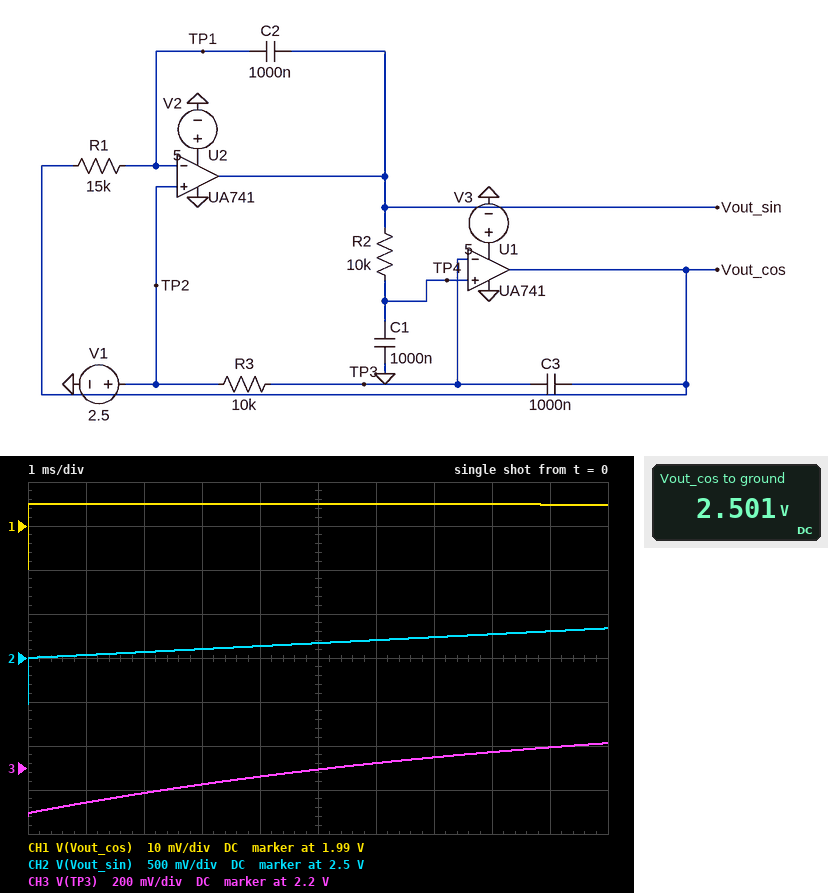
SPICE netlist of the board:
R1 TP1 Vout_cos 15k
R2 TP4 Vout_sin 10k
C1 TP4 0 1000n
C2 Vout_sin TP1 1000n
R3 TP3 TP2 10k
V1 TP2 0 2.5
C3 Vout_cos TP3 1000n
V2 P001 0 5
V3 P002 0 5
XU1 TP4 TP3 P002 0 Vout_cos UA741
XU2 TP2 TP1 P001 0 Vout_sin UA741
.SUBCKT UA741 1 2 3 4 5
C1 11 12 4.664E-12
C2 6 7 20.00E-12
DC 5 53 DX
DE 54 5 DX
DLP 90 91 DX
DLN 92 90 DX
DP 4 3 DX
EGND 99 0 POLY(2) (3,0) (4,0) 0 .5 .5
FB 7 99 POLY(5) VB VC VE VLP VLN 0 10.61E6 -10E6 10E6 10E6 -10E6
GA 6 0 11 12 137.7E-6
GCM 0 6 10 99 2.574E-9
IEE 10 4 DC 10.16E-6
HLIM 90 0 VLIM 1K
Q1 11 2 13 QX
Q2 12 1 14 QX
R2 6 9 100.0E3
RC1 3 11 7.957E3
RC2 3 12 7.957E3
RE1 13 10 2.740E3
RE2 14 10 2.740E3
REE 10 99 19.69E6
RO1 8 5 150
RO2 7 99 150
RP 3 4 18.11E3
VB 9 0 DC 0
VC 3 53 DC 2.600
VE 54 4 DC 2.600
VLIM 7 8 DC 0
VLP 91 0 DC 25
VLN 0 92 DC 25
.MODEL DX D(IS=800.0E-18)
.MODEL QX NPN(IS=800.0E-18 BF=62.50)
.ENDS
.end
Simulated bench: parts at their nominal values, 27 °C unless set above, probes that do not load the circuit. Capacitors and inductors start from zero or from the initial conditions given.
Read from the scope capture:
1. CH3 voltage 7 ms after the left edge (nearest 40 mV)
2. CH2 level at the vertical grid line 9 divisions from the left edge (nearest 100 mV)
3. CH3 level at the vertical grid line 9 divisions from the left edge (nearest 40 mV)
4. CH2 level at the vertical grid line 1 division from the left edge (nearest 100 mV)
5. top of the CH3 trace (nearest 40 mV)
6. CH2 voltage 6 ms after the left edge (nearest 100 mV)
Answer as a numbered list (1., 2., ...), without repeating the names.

1. 2.24 V
2. 2.8 V
3. 2.28 V
4. 2.5 V
5. 2.32 V
6. 2.7 V
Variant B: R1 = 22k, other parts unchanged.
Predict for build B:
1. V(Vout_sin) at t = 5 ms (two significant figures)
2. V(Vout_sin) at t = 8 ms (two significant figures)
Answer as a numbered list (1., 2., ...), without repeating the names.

1. 2.6 V
2. 2.7 V
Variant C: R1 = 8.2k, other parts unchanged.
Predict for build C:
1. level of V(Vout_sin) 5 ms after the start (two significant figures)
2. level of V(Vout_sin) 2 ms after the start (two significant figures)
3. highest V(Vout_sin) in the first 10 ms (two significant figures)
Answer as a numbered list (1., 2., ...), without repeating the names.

1. 2.8 V
2. 2.6 V
3. 3.0 V
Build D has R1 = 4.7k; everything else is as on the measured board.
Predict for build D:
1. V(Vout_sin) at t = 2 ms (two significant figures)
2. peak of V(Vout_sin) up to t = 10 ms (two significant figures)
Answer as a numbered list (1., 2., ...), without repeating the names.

1. 2.7 V
2. 3.0 V
